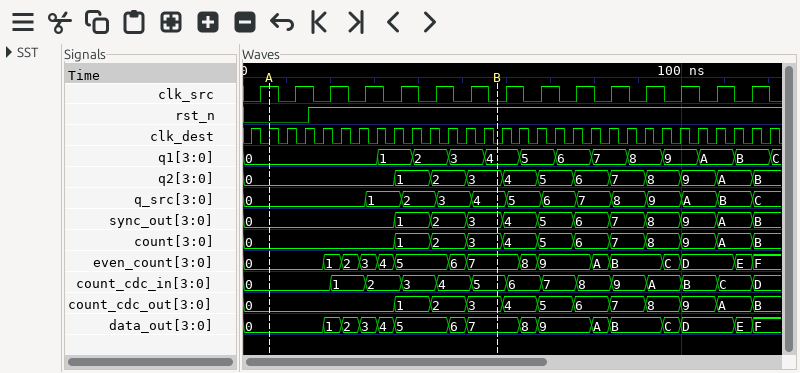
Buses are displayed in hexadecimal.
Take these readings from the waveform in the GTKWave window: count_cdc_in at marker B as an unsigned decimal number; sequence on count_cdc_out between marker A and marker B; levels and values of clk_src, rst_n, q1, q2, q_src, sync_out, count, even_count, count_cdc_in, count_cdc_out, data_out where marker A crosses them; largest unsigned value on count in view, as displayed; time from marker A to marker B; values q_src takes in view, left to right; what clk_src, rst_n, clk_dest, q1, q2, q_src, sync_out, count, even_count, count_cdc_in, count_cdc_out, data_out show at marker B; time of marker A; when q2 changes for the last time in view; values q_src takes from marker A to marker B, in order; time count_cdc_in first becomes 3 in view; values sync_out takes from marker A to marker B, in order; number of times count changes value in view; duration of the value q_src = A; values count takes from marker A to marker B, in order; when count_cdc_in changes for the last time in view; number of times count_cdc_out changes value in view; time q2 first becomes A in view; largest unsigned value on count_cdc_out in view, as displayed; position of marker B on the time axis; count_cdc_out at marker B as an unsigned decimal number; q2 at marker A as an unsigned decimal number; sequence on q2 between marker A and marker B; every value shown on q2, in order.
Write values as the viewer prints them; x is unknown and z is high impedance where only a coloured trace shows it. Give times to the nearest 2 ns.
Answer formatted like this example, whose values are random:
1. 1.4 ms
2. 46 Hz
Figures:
1. 5
2. 0, 1, 2, 3
3. clk_src=1, rst_n=0, q1=0, q2=0, q_src=0, sync_out=0, count=0, even_count=0, count_cdc_in=0, count_cdc_out=0, data_out=0
4. B
5. 52 ns
6. 0, 1, 2, 3, 4, 5, 6, 7, 8, 9, A, B, C
7. clk_src=0, rst_n=1, clk_dest=0, q1=4, q2=3, q_src=4, sync_out=3, count=3, even_count=7, count_cdc_in=5, count_cdc_out=3, data_out=7
8. 6 ns
9. 116 ns
10. 0, 1, 2, 3, 4
11. 36 ns
12. 0, 1, 2, 3
13. 11
14. 8 ns
15. 0, 1, 2, 3
16. 116 ns
17. 11
18. 108 ns
19. B
20. 58 ns
21. 3
22. 0
23. 0, 1, 2, 3
24. 0, 1, 2, 3, 4, 5, 6, 7, 8, 9, A, B
